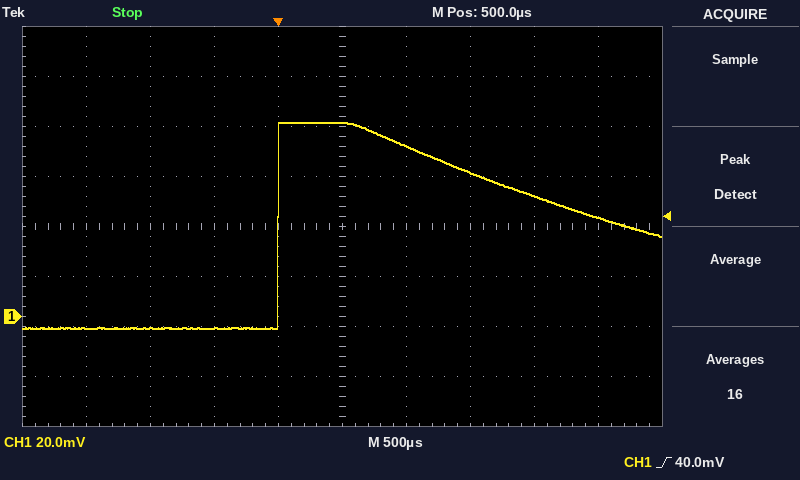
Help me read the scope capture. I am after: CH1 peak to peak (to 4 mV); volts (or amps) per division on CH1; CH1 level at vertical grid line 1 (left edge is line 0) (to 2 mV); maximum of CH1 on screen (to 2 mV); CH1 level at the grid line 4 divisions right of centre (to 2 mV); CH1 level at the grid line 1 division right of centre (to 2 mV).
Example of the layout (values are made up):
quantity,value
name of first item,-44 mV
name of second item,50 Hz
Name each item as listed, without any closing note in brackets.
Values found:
quantity,value
CH1 peak to peak,84 mV
volts (or amps) per division on CH1,20 mV
CH1 level at vertical grid line 1 (left edge is line 0),-4 mV
maximum of CH1 on screen,78 mV
CH1 level at the grid line 4 divisions right of centre,40 mV
CH1 level at the grid line 1 division right of centre,68 mV
